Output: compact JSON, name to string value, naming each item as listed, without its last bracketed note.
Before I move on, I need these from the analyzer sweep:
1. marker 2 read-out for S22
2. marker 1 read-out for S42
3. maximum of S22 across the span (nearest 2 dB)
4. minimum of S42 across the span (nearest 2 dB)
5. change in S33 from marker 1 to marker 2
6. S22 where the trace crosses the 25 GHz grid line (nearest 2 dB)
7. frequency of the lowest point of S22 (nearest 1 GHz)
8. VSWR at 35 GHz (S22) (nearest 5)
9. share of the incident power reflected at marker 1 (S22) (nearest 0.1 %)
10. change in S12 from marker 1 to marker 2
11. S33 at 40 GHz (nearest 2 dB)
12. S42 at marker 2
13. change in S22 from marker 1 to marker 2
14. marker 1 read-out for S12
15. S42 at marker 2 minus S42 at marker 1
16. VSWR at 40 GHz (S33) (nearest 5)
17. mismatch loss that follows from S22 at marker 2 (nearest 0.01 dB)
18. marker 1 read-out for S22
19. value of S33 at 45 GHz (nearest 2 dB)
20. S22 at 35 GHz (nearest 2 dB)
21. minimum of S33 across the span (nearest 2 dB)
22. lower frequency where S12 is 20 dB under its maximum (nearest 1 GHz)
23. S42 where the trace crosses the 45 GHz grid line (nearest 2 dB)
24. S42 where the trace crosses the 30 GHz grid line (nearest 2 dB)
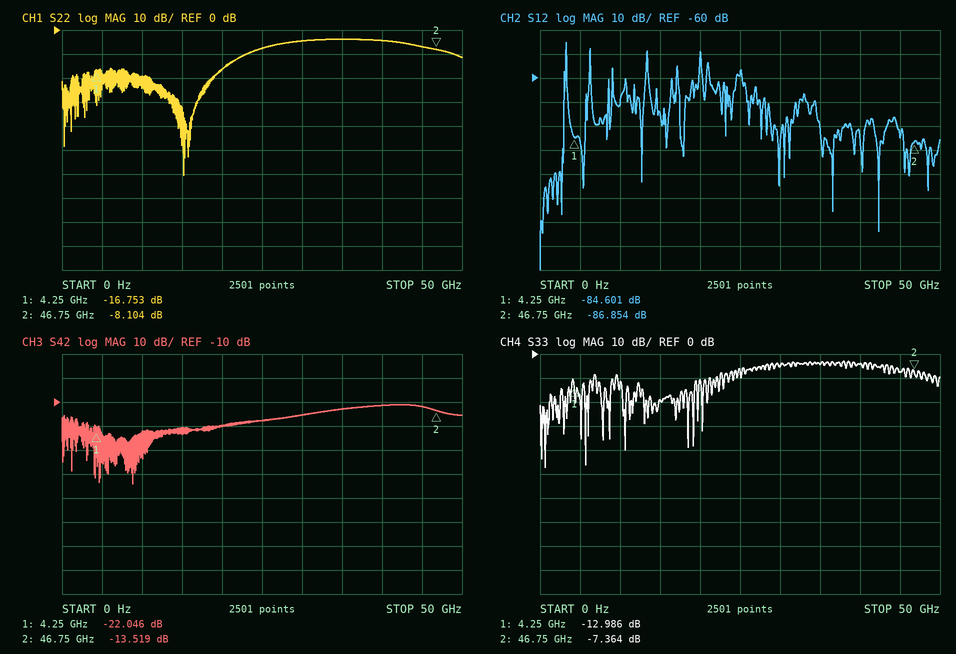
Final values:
{"marker 2 read-out for S22": "-8.104 dB", "marker 1 read-out for S42": "-22.046 dB", "maximum of S22 across the span": "-4 dB", "minimum of S42 across the span": "-44 dB", "change in S33 from marker 1 to marker 2": "5.622 dB", "S22 where the trace crosses the 25 GHz grid line": "-8 dB", "frequency of the lowest point of S22": "15 GHz", "VSWR at 35 GHz (S22)": "5", "share of the incident power reflected at marker 1 (S22)": "2.1 %", "change in S12 from marker 1 to marker 2": "-2.253 dB", "S33 at 40 GHz": "-4 dB", "S42 at marker 2": "-13.519 dB", "change in S22 from marker 1 to marker 2": "8.649 dB", "marker 1 read-out for S12": "-84.601 dB", "S42 at marker 2 minus S42 at marker 1": "8.527 dB", "VSWR at 40 GHz (S33)": "5", "mismatch loss that follows from S22 at marker 2": "0.73 dB", "marker 1 read-out for S22": "-16.753 dB", "value of S33 at 45 GHz": "-8 dB", "S22 at 35 GHz": "-4 dB", "minimum of S33 across the span": "-48 dB", "lower frequency where S12 is 20 dB under its maximum": "3 GHz", "S42 where the trace crosses the 45 GHz grid line": "-12 dB", "S42 where the trace crosses the 30 GHz grid line": "-16 dB"}
